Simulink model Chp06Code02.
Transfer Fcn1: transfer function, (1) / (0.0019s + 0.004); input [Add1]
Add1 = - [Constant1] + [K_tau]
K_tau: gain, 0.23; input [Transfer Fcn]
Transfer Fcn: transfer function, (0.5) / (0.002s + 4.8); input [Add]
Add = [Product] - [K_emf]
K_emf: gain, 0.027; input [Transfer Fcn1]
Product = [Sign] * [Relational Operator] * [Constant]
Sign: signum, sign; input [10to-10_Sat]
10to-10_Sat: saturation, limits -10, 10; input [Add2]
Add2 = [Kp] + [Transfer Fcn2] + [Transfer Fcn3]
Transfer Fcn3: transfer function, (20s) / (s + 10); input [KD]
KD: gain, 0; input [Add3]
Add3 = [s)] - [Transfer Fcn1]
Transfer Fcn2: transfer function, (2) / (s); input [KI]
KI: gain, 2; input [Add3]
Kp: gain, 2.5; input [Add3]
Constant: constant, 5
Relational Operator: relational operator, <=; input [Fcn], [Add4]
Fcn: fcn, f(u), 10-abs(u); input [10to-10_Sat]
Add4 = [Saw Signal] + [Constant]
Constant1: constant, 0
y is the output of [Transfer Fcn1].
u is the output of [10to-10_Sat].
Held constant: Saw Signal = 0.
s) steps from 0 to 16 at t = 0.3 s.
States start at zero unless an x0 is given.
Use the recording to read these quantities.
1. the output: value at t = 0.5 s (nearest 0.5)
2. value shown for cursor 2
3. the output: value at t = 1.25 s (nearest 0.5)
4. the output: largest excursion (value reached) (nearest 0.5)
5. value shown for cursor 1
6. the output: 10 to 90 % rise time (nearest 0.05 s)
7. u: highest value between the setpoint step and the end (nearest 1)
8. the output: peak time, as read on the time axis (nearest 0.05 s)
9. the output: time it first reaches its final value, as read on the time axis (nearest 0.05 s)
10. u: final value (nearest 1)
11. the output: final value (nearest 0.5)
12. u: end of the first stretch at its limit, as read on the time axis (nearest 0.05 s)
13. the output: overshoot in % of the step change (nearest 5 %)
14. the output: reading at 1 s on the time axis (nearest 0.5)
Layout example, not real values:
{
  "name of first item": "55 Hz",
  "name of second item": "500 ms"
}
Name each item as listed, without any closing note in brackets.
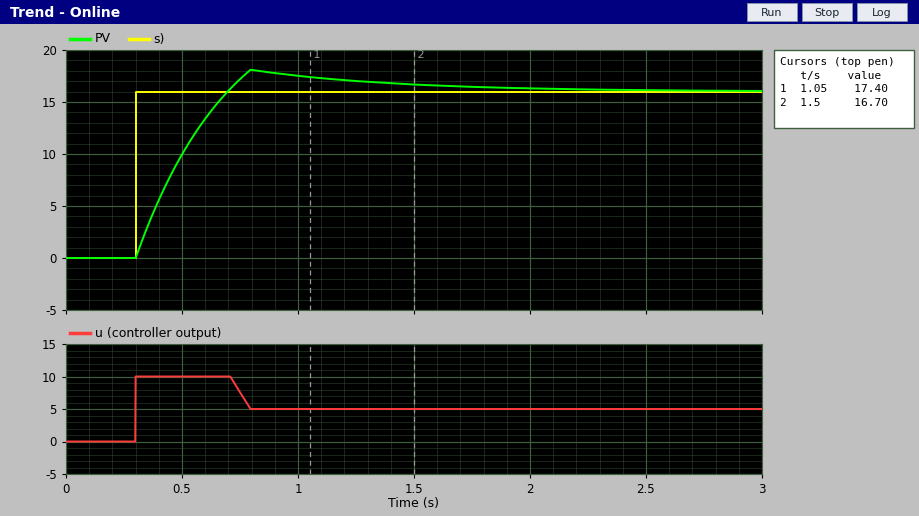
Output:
{
  "the output: value at t = 0.5 s": "10.0",
  "value shown for cursor 2": "16.70",
  "the output: value at t = 1.25 s": "17.0",
  "the output: largest excursion (value reached)": "18.0",
  "value shown for cursor 1": "17.40",
  "the output: 10 to 90 % rise time": "0.30 s",
  "u: highest value between the setpoint step and the end": "10",
  "the output: peak time, as read on the time axis": "0.80 s",
  "the output: time it first reaches its final value, as read on the time axis": "0.70 s",
  "u: final value": "5",
  "the output: final value": "16.0",
  "u: end of the first stretch at its limit, as read on the time axis": "0.70 s",
  "the output: overshoot in % of the step change": "15 %",
  "the output: reading at 1 s on the time axis": "17.5"
}
